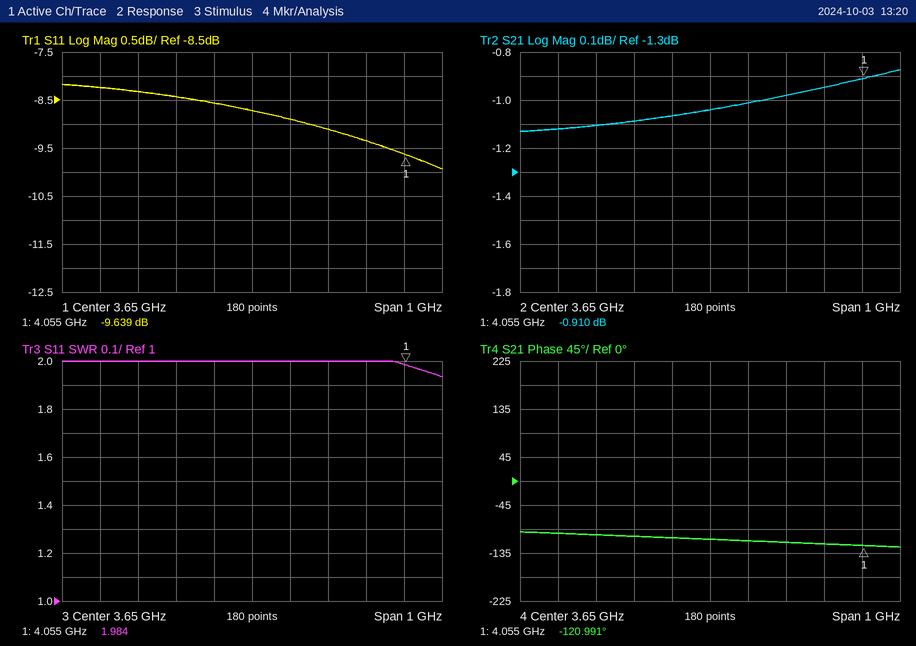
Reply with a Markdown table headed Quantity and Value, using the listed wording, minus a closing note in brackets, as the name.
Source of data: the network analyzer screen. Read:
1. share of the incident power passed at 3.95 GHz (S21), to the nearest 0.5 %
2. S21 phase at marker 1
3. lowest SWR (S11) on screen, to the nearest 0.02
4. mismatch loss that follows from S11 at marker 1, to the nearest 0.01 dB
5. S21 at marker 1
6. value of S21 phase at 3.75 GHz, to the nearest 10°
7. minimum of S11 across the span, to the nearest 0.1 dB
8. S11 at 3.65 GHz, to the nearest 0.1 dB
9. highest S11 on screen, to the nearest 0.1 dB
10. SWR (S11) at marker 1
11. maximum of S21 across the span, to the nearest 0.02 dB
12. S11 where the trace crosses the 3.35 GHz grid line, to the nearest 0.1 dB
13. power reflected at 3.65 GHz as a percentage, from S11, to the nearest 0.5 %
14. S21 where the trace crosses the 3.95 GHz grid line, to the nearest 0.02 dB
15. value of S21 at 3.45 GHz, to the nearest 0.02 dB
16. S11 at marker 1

| Quantity | Value |
|---|---|
| share of the incident power passed at 3.95 GHz (S21), to the nearest 0.5 % | 80.5 % |
| S21 phase at marker 1 | -120.991° |
| lowest SWR (S11) on screen, to the nearest 0.02 | 1.94 |
| mismatch loss that follows from S11 at marker 1, to the nearest 0.01 dB | 0.50 dB |
| S21 at marker 1 | -0.910 dB |
| value of S21 phase at 3.75 GHz, to the nearest 10° | -110° |
| minimum of S11 across the span, to the nearest 0.1 dB | -9.9 dB |
| S11 at 3.65 GHz, to the nearest 0.1 dB | -8.7 dB |
| highest S11 on screen, to the nearest 0.1 dB | -8.2 dB |
| SWR (S11) at marker 1 | 1.984 |
| maximum of S21 across the span, to the nearest 0.02 dB | -0.88 dB |
| S11 where the trace crosses the 3.35 GHz grid line, to the nearest 0.1 dB | -8.3 dB |
| power reflected at 3.65 GHz as a percentage, from S11, to the nearest 0.5 % | 13.5 % |
| S21 where the trace crosses the 3.95 GHz grid line, to the nearest 0.02 dB | -0.94 dB |
| value of S21 at 3.45 GHz, to the nearest 0.02 dB | -1.08 dB |
| S11 at marker 1 | -9.639 dB |
